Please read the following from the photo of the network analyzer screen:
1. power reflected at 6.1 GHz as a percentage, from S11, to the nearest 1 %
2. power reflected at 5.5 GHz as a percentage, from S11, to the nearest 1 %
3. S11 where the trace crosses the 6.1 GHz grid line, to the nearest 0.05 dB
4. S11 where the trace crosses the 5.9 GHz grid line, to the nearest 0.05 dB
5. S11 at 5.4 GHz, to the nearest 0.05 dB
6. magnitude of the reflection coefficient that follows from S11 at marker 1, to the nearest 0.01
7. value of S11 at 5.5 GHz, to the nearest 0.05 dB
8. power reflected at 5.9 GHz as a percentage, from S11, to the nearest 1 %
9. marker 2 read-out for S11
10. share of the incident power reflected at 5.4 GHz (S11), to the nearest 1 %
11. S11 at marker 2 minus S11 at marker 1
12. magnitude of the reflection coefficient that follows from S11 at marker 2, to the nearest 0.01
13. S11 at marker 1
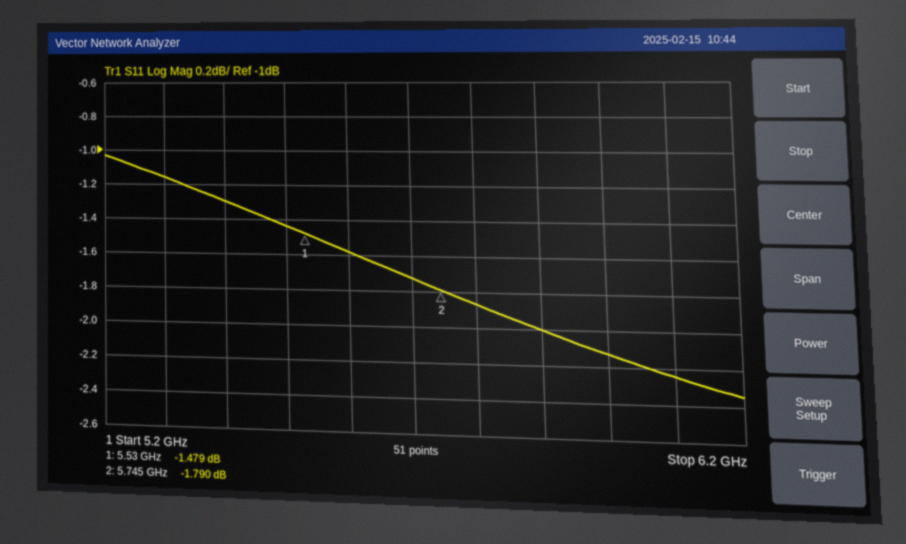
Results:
60 %
72 %
-2.25 dB
-2.00 dB
-1.30 dB
0.84
-1.45 dB
63 %
-1.790 dB
74 %
-0.311 dB
0.81
-1.479 dB
